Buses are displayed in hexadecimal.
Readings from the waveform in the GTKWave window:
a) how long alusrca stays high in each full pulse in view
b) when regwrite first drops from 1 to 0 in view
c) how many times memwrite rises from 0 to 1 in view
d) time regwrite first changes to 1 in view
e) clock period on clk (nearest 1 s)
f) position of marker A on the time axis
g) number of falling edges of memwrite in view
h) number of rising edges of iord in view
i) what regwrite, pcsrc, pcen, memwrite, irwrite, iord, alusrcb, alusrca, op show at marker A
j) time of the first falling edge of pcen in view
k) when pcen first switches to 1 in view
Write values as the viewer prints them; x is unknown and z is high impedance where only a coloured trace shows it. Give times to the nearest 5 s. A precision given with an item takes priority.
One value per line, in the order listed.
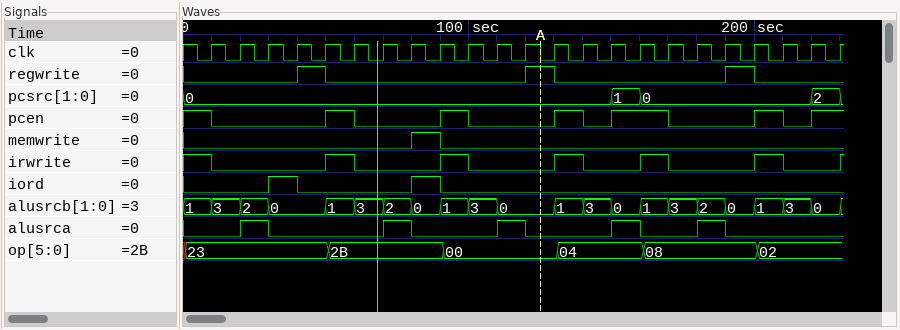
10 s, 10 s, 10 s, 10 s, 10 s
50 s
1
40 s
10 s
125 s
1
2
regwrite=1, pcsrc=0, pcen=0, memwrite=0, irwrite=0, iord=0, alusrcb=0, alusrca=0, op=00
10 s
50 s
